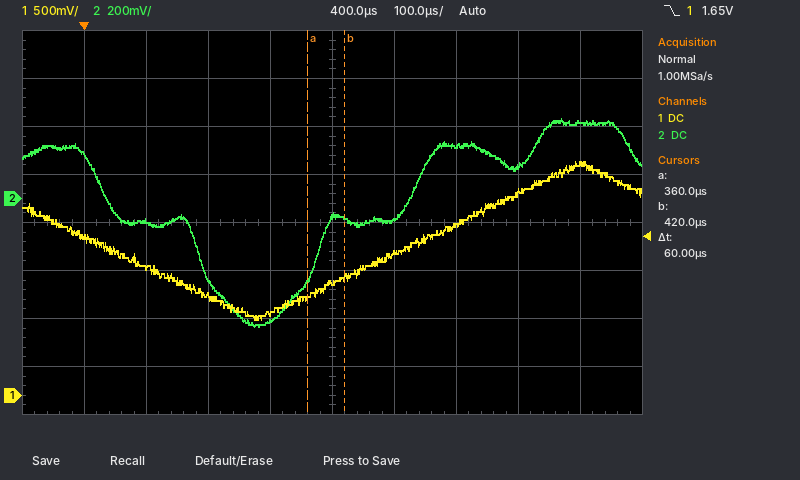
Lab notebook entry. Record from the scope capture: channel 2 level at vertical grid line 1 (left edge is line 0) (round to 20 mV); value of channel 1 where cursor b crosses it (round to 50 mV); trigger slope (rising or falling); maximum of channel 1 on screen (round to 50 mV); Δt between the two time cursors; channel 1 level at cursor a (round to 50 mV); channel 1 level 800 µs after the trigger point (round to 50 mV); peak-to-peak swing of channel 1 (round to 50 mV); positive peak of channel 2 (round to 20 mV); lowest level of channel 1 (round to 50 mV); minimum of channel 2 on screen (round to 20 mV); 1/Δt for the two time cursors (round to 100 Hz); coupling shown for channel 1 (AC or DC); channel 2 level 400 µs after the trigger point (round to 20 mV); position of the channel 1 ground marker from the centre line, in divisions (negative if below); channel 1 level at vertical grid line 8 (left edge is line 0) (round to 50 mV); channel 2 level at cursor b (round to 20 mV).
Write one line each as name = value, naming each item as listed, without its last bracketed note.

channel 2 level at vertical grid line 1 (left edge is line 0) = 180 mV
value of channel 1 where cursor b crosses it = 1.25 V
trigger slope = falling
maximum of channel 1 on screen = 2.45 V
Δt between the two time cursors = 60 µs
channel 1 level at cursor a = 1.05 V
channel 1 level 800 µs after the trigger point = 2.40 V
peak-to-peak swing of channel 1 = 1.65 V
positive peak of channel 2 = 340 mV
lowest level of channel 1 = 800 mV
minimum of channel 2 on screen = -540 mV
1/Δt for the two time cursors = 16.7 kHz
coupling shown for channel 1 = DC
channel 2 level 400 µs after the trigger point = -80 mV
position of the channel 1 ground marker from the centre line, in divisions = -3.6 div
channel 1 level at vertical grid line 8 (left edge is line 0) = 2.10 V
channel 2 level at cursor b = -80 mV
